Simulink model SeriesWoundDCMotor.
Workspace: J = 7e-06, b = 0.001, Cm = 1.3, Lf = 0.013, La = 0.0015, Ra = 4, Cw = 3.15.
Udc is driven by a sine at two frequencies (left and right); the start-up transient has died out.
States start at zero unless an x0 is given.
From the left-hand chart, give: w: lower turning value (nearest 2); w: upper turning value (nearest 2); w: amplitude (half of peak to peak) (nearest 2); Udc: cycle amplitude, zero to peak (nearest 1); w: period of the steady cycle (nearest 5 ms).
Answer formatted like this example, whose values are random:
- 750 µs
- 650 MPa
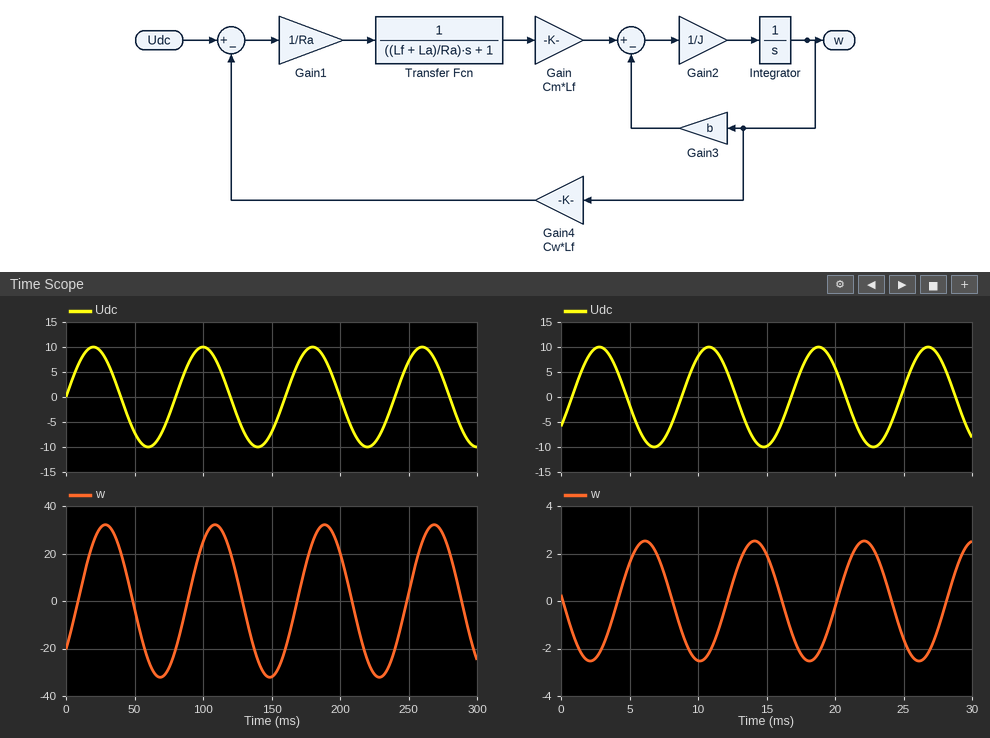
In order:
- -32
- 32
- 32
- 10
- 80 ms
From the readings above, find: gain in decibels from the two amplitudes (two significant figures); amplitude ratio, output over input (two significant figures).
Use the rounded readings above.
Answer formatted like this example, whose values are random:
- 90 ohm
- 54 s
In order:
- 10 dB
- 3.2
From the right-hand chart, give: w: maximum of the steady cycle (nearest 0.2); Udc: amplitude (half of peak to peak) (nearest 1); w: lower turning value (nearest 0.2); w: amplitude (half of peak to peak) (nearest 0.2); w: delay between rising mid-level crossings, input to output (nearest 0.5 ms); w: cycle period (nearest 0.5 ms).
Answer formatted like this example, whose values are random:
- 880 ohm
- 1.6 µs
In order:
- 2.6
- 10
- -2.6
- 2.6
- 3.5 ms
- 8.0 ms
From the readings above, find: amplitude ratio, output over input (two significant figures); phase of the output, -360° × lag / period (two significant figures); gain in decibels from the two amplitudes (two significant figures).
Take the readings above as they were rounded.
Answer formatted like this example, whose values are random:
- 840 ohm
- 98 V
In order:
- 0.26
- -160°
- -12 dB
